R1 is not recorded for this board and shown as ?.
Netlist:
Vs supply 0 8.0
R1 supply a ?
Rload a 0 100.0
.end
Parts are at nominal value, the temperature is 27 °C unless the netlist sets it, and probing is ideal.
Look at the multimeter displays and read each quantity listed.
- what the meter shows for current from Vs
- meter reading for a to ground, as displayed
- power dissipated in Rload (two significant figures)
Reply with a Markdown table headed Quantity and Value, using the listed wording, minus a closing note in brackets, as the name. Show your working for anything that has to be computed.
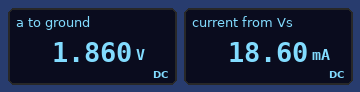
| Quantity | Value |
|---|---|
| what the meter shows for current from Vs | 18.60 mA |
| meter reading for a to ground, as displayed | 1.860 V |
| power dissipated in Rload | (1.86 V)^2 / 100 Ω = 35 mW |
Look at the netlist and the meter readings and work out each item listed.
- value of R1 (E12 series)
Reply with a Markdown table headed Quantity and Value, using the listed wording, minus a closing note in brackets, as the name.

| Quantity | Value |
|---|---|
| value of R1 | 330 Ω |
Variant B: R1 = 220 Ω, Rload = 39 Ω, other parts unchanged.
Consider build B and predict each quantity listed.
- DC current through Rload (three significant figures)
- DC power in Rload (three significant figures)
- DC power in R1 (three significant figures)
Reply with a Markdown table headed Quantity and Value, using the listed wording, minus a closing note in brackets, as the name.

| Quantity | Value |
|---|---|
| DC current through Rload | 30.9 mA |
| DC power in Rload | 37.2 mW |
| DC power in R1 | 210 mW |
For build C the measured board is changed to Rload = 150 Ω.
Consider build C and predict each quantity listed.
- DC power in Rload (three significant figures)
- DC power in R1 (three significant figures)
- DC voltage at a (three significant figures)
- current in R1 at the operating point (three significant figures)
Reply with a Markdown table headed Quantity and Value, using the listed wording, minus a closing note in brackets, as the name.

| Quantity | Value |
|---|---|
| DC power in Rload | 41.7 mW |
| DC power in R1 | 91.7 mW |
| DC voltage at a | 2.50 V |
| current in R1 at the operating point | 16.7 mA |
